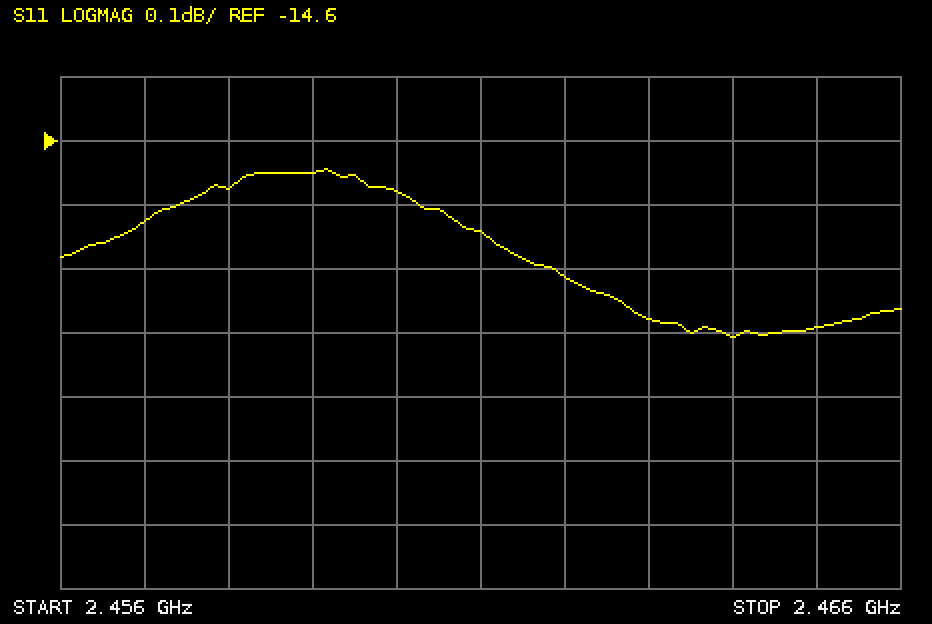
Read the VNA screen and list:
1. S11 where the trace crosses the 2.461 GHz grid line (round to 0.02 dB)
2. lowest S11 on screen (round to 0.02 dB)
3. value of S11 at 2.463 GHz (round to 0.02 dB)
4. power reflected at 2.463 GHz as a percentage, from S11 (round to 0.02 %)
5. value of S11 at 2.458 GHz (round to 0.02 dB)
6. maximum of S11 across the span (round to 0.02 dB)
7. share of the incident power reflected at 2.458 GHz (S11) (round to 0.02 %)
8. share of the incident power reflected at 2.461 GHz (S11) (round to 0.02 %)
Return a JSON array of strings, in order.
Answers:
["-14.74 dB", "-14.90 dB", "-14.88 dB", "3.26 %", "-14.68 dB", "-14.64 dB", "3.40 %", "3.36 %"]
